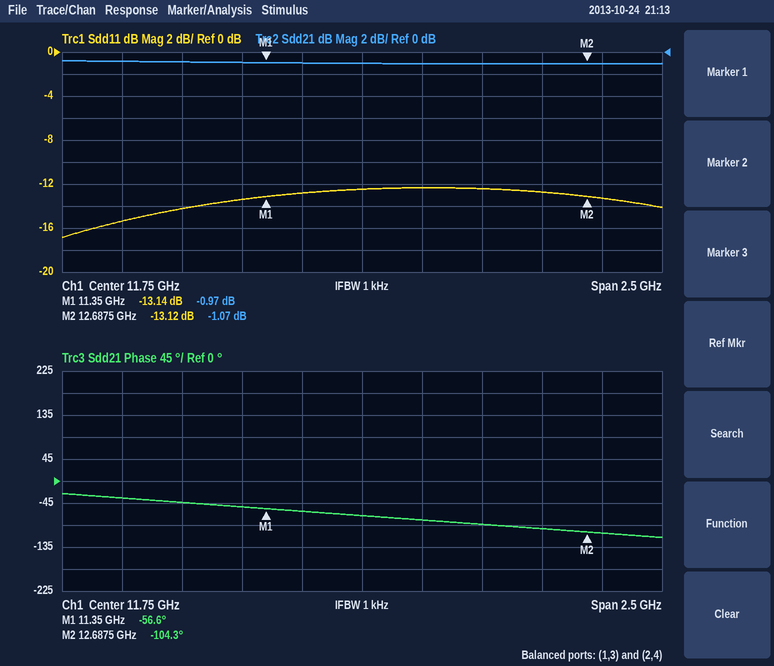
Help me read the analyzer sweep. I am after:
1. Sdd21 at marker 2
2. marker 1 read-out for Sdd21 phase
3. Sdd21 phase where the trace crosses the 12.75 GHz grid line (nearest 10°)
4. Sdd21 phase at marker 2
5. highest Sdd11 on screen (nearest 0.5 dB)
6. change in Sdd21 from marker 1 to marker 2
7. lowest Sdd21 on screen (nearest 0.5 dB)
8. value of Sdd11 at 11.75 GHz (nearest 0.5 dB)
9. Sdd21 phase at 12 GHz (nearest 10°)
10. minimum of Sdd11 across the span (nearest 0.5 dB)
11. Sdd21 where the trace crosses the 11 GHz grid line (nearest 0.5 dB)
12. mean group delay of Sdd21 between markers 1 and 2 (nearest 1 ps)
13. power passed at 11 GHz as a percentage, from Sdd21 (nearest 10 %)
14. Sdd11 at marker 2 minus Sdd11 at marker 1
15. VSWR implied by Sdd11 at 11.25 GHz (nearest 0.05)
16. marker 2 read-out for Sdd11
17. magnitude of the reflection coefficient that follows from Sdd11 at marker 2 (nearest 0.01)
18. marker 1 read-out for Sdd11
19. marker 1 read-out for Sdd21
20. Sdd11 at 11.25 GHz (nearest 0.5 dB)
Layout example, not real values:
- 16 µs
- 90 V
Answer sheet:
- -1.07 dB
- -56.6°
- -110°
- -104.3°
- -12.5 dB
- -0.10 dB
- -1.0 dB
- -12.5 dB
- -80°
- -17.0 dB
- -1.0 dB
- 99 ps
- 80 %
- 0.02 dB
- 1.55
- -13.12 dB
- 0.22
- -13.14 dB
- -0.97 dB
- -13.5 dB
